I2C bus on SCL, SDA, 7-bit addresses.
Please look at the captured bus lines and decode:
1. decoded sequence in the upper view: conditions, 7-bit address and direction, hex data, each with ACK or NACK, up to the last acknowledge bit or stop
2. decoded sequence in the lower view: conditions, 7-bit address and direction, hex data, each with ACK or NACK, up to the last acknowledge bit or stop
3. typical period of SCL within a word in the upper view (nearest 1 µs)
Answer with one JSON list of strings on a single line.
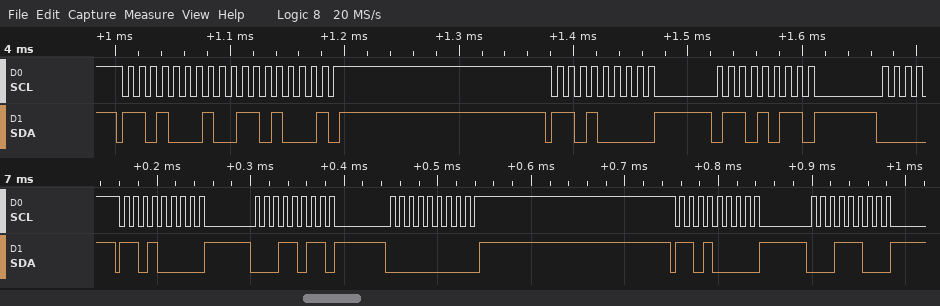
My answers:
["start, address 68 read ACK, 68 NACK, stop, start, address 68 write ACK, 6B ACK", "start, address 68 write ACK, 1B ACK, 00 ACK, stop, start, address 68 write ACK, 1C ACK", "10 µs"]
